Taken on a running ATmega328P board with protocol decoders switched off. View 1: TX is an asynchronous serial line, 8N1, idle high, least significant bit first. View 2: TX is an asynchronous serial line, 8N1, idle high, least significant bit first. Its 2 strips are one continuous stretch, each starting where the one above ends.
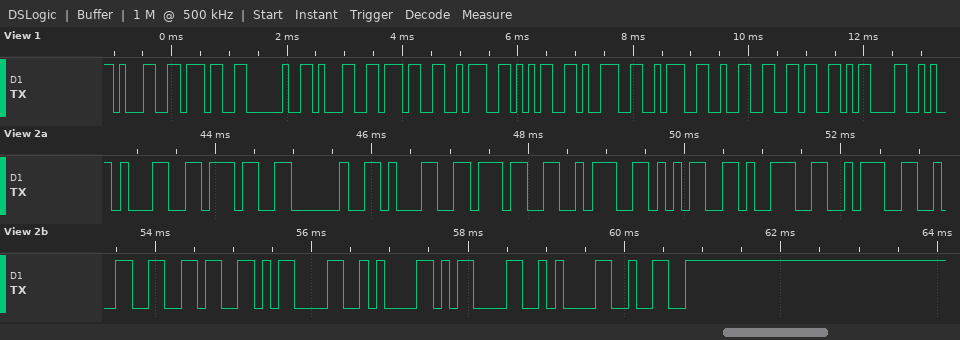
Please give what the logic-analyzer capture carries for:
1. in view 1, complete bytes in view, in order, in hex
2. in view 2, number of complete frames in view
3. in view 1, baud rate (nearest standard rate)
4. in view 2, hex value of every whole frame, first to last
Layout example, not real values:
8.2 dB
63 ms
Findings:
31 37 20 31 37 3A 35 39 3A 32 36 0D
16
9600 baud
0x31 0x37 0x20 0x31 0x37 0x3A 0x35 0x39 0x3A 0x32 0x36 0x0D 0x0A 0x0D 0x0A 0x32
